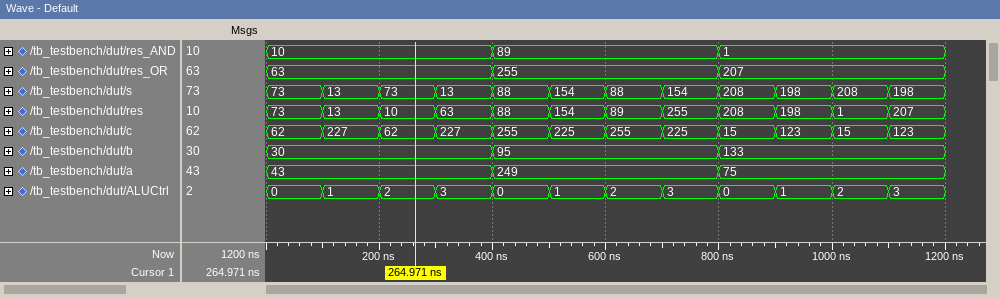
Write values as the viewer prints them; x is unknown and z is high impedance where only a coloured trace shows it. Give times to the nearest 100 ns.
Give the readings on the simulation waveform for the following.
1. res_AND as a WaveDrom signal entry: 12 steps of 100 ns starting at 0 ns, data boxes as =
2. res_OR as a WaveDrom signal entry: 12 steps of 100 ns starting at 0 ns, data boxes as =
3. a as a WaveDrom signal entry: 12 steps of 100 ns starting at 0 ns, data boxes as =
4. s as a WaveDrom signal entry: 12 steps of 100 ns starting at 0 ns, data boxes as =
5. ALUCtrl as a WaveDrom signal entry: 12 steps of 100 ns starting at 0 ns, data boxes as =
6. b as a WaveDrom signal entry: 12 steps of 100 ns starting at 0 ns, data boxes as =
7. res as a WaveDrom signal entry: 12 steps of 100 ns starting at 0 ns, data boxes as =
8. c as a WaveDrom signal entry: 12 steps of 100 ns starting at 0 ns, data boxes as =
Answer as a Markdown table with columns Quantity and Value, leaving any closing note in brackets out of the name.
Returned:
| Quantity | Value |
|---|---|
| res_AND as a WaveDrom signal entry: 12 steps of 100 ns starting at 0 ns, data boxes as = | {name: 'res_AND', wave: '=...=...=...', data: '10 89 1'} |
| res_OR as a WaveDrom signal entry: 12 steps of 100 ns starting at 0 ns, data boxes as = | {name: 'res_OR', wave: '=...=...=...', data: '63 255 207'} |
| a as a WaveDrom signal entry: 12 steps of 100 ns starting at 0 ns, data boxes as = | {name: 'a', wave: '=...=...=...', data: '43 249 75'} |
| s as a WaveDrom signal entry: 12 steps of 100 ns starting at 0 ns, data boxes as = | {name: 's', wave: '============', data: '73 13 73 13 88 154 88 154 208 198 208 198'} |
| ALUCtrl as a WaveDrom signal entry: 12 steps of 100 ns starting at 0 ns, data boxes as = | {name: 'ALUCtrl', wave: '============', data: '0 1 2 3 0 1 2 3 0 1 2 3'} |
| b as a WaveDrom signal entry: 12 steps of 100 ns starting at 0 ns, data boxes as = | {name: 'b', wave: '=...=...=...', data: '30 95 133'} |
| res as a WaveDrom signal entry: 12 steps of 100 ns starting at 0 ns, data boxes as = | {name: 'res', wave: '============', data: '73 13 10 63 88 154 89 255 208 198 1 207'} |
| c as a WaveDrom signal entry: 12 steps of 100 ns starting at 0 ns, data boxes as = | {name: 'c', wave: '============', data: '62 227 62 227 255 225 255 225 15 123 15 123'} |
